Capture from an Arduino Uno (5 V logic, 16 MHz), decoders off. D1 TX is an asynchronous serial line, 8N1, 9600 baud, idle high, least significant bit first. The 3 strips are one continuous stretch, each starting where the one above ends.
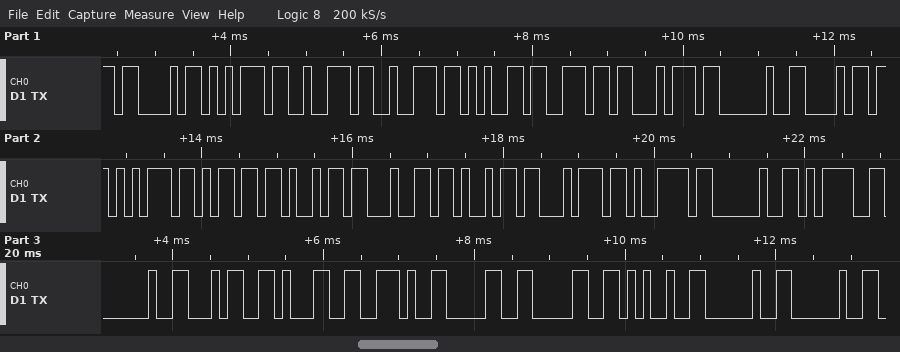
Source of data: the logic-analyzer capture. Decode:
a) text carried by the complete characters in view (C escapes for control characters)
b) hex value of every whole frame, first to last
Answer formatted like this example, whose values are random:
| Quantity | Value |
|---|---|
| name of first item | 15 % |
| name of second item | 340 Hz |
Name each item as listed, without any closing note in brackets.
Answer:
| Quantity | Value |
|---|---|
| text carried by the complete characters in view | "Current humidity = 41.00%  " |
| hex value of every whole frame, first to last | 43 75 72 72 65 6E 74 20 68 75 6D 69 64 69 74 79 20 3D 20 34 31 2E 30 30 25 20 20 |
